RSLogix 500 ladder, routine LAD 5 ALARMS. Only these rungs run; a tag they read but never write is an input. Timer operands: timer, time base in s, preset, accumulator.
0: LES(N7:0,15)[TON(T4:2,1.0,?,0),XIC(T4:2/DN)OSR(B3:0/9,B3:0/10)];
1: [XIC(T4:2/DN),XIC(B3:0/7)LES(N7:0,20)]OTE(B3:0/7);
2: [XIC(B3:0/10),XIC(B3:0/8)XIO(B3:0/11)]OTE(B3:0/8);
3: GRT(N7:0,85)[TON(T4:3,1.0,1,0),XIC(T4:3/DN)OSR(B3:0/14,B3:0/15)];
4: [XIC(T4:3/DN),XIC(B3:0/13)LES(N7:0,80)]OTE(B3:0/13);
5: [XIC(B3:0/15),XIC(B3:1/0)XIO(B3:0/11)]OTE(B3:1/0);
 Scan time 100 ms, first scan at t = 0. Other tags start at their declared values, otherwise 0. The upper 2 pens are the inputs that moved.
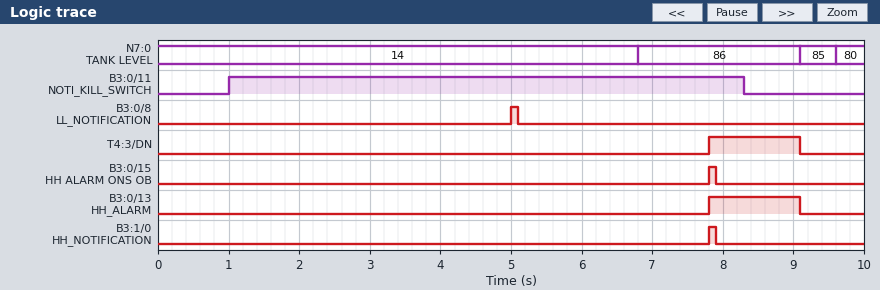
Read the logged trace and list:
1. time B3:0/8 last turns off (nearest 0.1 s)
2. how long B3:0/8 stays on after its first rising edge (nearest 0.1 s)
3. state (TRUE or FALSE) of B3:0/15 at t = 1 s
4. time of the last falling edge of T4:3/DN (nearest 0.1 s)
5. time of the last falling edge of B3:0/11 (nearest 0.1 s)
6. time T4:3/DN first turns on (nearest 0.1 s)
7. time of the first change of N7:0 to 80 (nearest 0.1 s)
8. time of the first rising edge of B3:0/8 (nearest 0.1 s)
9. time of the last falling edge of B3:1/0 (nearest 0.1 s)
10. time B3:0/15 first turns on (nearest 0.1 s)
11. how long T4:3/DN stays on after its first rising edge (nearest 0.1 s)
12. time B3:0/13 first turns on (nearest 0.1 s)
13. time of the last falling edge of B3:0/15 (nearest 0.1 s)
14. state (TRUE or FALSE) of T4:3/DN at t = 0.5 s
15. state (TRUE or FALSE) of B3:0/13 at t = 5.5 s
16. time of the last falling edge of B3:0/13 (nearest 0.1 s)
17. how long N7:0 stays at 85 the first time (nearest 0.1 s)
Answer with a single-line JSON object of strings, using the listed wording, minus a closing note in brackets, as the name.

{"time B3:0/8 last turns off": "5.1 s", "how long B3:0/8 stays on after its first rising edge": "0.1 s", "state (TRUE or FALSE) of B3:0/15 at t = 1 s": "FALSE", "time of the last falling edge of T4:3/DN": "9.1 s", "time of the last falling edge of B3:0/11": "8.3 s", "time T4:3/DN first turns on": "7.8 s", "time of the first change of N7:0 to 80": "9.6 s", "time of the first rising edge of B3:0/8": "5.0 s", "time of the last falling edge of B3:1/0": "7.9 s", "time B3:0/15 first turns on": "7.8 s", "how long T4:3/DN stays on after its first rising edge": "1.3 s", "time B3:0/13 first turns on": "7.8 s", "time of the last falling edge of B3:0/15": "7.9 s", "state (TRUE or FALSE) of T4:3/DN at t = 0.5 s": "FALSE", "state (TRUE or FALSE) of B3:0/13 at t = 5.5 s": "FALSE", "time of the last falling edge of B3:0/13": "9.1 s", "how long N7:0 stays at 85 the first time": "0.5 s"}
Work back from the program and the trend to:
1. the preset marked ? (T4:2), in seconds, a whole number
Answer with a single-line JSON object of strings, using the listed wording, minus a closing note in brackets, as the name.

{"the preset marked ? (T4:2), in seconds, a whole number": "5 s"}
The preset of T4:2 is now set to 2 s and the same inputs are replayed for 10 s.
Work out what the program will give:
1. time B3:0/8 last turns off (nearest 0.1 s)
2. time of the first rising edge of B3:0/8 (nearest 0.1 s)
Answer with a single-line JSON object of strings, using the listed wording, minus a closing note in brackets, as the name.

{"time B3:0/8 last turns off": "2.1 s", "time of the first rising edge of B3:0/8": "2.0 s"}
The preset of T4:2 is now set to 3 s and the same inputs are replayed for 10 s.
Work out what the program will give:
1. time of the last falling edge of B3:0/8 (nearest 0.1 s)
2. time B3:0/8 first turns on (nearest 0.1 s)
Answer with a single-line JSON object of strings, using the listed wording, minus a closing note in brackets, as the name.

{"time of the last falling edge of B3:0/8": "3.1 s", "time B3:0/8 first turns on": "3.0 s"}
